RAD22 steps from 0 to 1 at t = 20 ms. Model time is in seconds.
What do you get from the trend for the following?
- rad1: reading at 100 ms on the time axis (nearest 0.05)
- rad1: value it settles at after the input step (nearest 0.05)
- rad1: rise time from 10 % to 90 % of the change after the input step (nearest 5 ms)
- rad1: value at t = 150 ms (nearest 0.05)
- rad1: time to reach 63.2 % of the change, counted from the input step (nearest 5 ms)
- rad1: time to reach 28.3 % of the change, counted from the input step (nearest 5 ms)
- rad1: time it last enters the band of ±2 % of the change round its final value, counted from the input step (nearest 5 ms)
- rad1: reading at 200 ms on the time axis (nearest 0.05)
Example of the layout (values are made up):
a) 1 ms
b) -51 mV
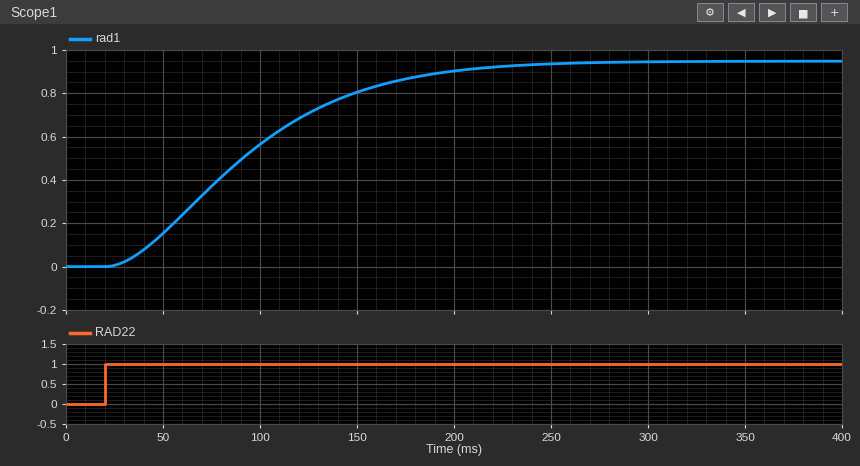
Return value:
a) 0.55
b) 0.95
c) 125 ms
d) 0.80
e) 85 ms
f) 45 ms
g) 215 ms
h) 0.90
